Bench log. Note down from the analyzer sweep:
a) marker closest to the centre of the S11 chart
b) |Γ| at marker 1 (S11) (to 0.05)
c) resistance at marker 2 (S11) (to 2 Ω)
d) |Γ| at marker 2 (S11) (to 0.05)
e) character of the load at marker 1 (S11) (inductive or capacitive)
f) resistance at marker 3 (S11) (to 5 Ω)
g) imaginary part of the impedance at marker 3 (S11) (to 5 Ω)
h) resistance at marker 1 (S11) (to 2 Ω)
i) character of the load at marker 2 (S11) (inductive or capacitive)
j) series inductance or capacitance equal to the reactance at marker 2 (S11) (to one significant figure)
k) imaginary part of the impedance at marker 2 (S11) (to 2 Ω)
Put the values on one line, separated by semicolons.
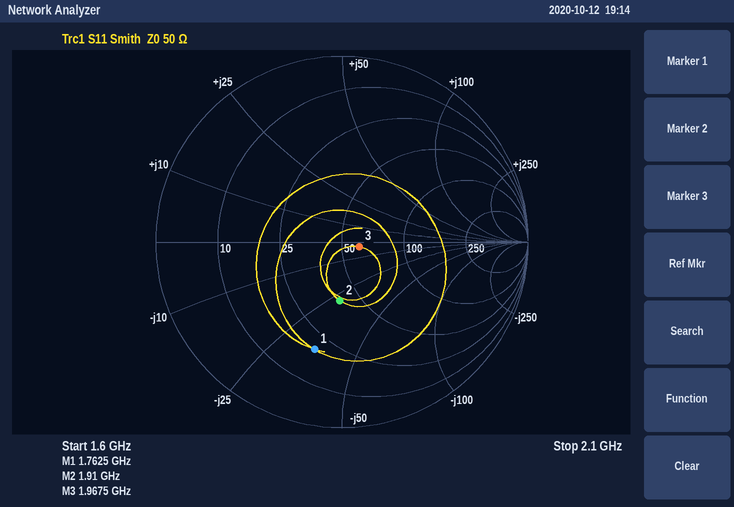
marker 3; 0.60; 40 Ω; 0.30; capacitive; 60 Ω; -5 Ω; 20 Ω; capacitive; 3 pF; -28 Ω
